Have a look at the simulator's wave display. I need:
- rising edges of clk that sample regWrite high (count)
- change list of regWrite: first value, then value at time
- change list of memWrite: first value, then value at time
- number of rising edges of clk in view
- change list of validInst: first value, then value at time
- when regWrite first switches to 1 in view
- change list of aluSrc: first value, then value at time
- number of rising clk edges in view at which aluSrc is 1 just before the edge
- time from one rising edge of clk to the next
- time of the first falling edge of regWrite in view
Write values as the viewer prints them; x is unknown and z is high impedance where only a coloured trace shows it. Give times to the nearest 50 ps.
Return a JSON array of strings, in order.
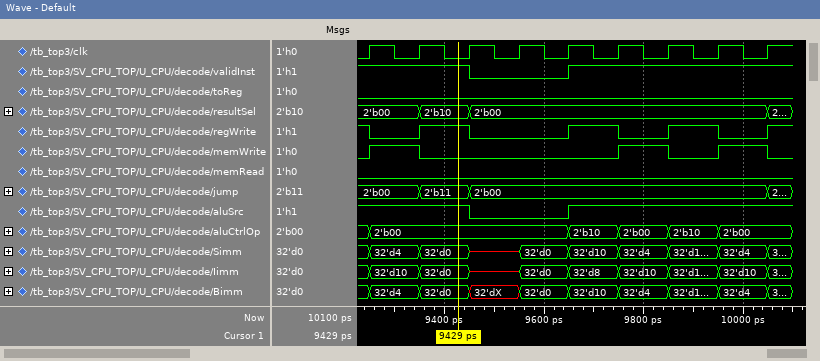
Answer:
["4", "1, 0 at 9250 ps, 1 at 9350 ps, 0 at 9450 ps, 1 at 9650 ps, 0 at 9750 ps, 1 at 9850 ps, 0 at 9950 ps, 1 at 10050 ps", "0, 1 at 9250 ps, 0 at 9350 ps, 1 at 9750 ps, 0 at 9850 ps, 1 at 9950 ps, 0 at 10050 ps", "9", "1, 0 at 9450 ps, 1 at 9650 ps", "9350 ps", "1, 0 at 9450 ps, 1 at 9650 ps", "7", "100 ps", "9250 ps"]
